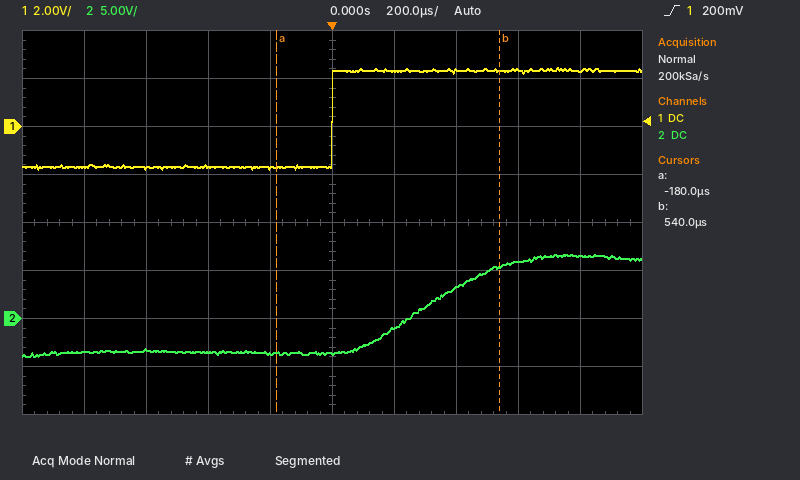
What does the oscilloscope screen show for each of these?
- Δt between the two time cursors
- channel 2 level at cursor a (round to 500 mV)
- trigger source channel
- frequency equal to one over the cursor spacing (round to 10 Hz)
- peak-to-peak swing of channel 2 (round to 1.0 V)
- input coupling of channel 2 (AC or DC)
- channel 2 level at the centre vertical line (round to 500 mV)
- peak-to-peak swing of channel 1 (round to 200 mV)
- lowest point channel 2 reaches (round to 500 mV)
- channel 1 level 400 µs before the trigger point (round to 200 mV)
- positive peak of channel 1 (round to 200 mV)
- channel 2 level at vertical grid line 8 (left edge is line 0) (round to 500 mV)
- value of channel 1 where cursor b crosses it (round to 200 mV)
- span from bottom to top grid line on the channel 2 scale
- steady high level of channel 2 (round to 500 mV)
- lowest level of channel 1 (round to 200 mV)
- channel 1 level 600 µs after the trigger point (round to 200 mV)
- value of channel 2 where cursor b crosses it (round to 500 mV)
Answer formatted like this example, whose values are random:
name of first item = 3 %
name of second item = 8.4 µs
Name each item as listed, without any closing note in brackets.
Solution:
Δt between the two time cursors = 720 µs
channel 2 level at cursor a = -3.5 V
trigger source channel = channel 1
frequency equal to one over the cursor spacing = 1.39 kHz
peak-to-peak swing of channel 2 = 11.0 V
input coupling of channel 2 = DC
channel 2 level at the centre vertical line = -3.5 V
peak-to-peak swing of channel 1 = 4.2 V
lowest point channel 2 reaches = -4.0 V
channel 1 level 400 µs before the trigger point = -1.6 V
positive peak of channel 1 = 2.4 V
channel 2 level at vertical grid line 8 (left edge is line 0) = 6.0 V
value of channel 1 where cursor b crosses it = 2.4 V
span from bottom to top grid line on the channel 2 scale = 40 V
steady high level of channel 2 = 6.5 V
lowest level of channel 1 = -1.8 V
channel 1 level 600 µs after the trigger point = 2.4 V
value of channel 2 where cursor b crosses it = 5.5 V
